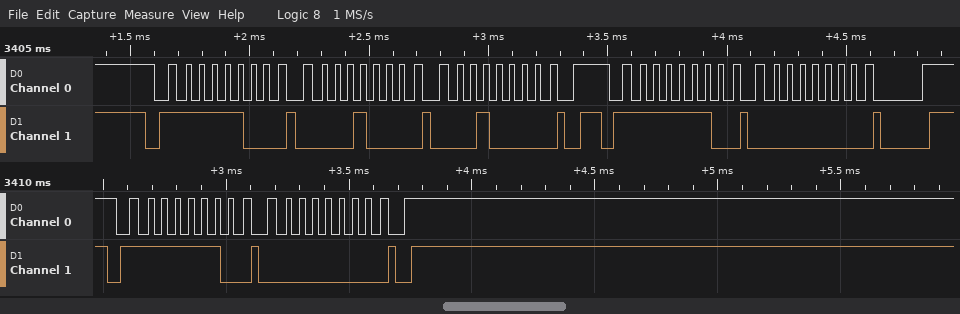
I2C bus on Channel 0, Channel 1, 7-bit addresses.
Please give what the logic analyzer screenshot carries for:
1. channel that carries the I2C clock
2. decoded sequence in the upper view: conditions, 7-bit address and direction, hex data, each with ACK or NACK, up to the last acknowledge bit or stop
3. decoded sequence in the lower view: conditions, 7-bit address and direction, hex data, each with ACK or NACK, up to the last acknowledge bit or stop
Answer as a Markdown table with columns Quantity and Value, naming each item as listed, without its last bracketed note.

| Quantity | Value |
|---|---|
| channel that carries the I2C clock | Channel 0 |
| decoded sequence in the upper view: conditions, 7-bit address and direction, hex data, each with ACK or NACK, up to the last acknowledge bit or stop | start, address 7E write ACK, 08 ACK, 10 ACK, stop, start, address 7F write ACK, 00 ACK, stop |
| decoded sequence in the lower view: conditions, 7-bit address and direction, hex data, each with ACK or NACK, up to the last acknowledge bit or stop | start, address 7F write ACK, 00 ACK, stop |
